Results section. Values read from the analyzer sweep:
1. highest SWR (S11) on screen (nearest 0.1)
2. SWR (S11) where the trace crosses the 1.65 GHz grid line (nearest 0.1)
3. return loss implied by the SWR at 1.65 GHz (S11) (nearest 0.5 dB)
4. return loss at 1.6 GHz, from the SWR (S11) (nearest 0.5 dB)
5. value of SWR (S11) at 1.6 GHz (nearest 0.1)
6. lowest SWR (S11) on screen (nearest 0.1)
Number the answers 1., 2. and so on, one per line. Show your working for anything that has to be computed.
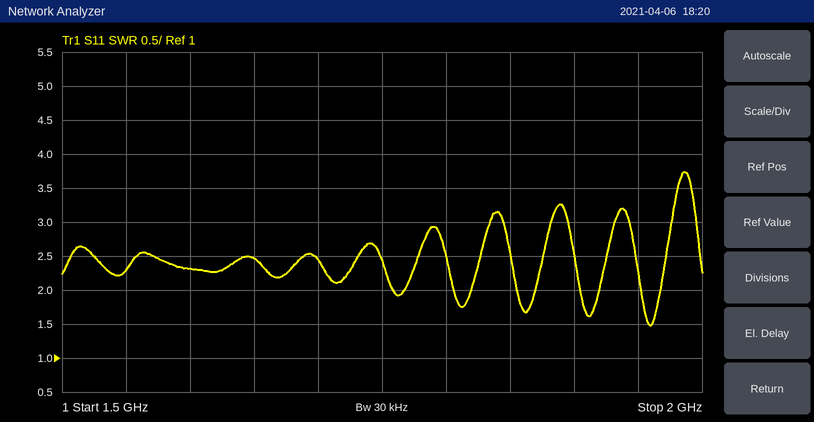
1. 3.7
2. 2.5
3. −20 log10((2.5 − 1)/(2.5 + 1)) ≈ 7.36 dB, so 7.5 dB to the nearest 0.5 dB
4. −20 log10((2.3 − 1)/(2.3 + 1)) ≈ 8.09 dB, so 8.0 dB to the nearest 0.5 dB
5. 2.3
6. 1.5
